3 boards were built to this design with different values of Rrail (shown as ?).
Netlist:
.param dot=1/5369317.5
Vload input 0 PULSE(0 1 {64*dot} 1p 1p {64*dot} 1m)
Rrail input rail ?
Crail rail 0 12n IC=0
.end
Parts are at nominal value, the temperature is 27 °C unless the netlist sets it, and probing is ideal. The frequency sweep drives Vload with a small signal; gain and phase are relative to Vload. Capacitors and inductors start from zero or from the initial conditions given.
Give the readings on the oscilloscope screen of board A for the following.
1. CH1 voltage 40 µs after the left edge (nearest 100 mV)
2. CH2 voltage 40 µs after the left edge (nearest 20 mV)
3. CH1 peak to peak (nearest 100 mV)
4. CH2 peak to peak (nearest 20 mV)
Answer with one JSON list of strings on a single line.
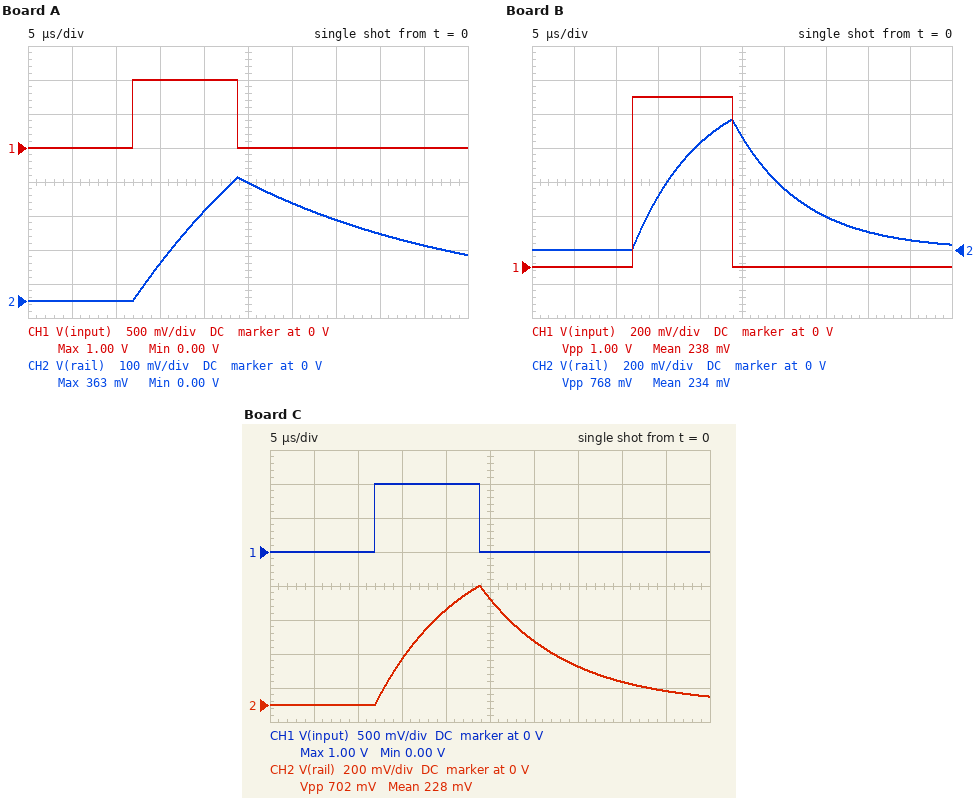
["0 V", "200 mV", "1.0 V", "360 mV"]
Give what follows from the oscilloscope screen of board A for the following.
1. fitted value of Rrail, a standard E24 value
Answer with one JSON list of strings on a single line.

["2.2 kΩ"]
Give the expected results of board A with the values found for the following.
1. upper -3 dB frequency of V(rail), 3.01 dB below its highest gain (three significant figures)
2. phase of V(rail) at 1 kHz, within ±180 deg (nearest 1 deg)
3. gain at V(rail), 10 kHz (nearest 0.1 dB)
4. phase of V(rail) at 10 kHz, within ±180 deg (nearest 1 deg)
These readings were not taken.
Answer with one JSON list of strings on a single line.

["6.03 kHz", "-9 deg", "-5.7 dB", "-59 deg"]
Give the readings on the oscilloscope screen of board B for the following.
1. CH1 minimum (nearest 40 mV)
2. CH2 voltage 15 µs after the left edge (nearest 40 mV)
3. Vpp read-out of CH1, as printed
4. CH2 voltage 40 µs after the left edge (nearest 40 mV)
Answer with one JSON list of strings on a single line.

["0 V", "320 mV", "1.00 V", "120 mV"]
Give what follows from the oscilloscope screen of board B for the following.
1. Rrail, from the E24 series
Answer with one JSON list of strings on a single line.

["680 Ω"]
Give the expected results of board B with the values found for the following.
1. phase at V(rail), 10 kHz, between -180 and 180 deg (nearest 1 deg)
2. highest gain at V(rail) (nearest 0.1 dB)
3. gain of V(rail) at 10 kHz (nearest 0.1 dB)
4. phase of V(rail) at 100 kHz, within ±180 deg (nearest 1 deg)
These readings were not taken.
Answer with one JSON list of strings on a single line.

["-27 deg", "0 dB", "-1.0 dB", "-79 deg"]
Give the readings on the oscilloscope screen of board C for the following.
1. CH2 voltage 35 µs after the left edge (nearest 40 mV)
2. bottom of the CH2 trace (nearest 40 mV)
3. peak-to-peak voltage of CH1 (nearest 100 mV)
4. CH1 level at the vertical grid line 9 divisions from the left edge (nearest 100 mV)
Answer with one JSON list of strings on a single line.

["240 mV", "0 V", "1.0 V", "0 V"]
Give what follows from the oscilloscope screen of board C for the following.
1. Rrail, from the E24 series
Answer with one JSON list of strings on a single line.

["820 Ω"]
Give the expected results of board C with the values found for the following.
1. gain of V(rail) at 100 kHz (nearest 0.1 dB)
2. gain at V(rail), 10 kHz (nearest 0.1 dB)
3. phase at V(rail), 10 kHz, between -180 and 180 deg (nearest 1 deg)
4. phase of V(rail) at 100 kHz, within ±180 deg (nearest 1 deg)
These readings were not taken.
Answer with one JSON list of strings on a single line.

["-15.9 dB", "-1.4 dB", "-32 deg", "-81 deg"]
